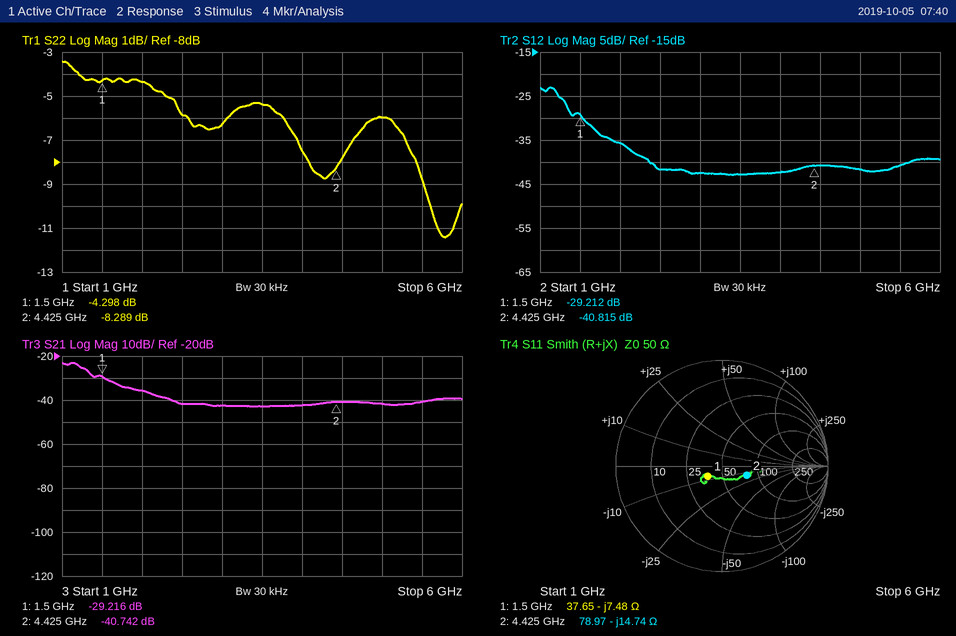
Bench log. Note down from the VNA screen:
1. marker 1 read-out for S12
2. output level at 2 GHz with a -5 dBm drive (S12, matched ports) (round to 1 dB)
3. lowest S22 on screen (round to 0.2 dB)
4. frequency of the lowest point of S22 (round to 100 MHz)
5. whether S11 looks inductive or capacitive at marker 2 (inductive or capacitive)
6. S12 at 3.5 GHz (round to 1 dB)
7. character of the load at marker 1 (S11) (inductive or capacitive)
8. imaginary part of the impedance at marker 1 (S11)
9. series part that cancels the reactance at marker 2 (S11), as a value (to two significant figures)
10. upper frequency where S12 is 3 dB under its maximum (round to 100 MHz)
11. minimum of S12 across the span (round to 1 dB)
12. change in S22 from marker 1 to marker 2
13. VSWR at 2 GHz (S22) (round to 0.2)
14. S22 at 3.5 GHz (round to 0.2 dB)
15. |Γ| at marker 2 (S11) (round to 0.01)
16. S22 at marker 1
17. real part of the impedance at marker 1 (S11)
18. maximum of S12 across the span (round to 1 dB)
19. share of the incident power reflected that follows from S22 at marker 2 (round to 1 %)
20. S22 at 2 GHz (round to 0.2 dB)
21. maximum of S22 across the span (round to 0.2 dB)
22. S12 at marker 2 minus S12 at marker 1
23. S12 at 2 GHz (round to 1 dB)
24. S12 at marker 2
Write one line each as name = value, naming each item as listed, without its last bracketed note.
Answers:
marker 1 read-out for S12 = -29.212 dB
output level at 2 GHz with a -5 dBm drive (S12, matched ports) = -41 dBm
lowest S22 on screen = -11.4 dB
frequency of the lowest point of S22 = 5.8 GHz
whether S11 looks inductive or capacitive at marker 2 = capacitive
S12 at 3.5 GHz = -43 dB
character of the load at marker 1 (S11) = capacitive
imaginary part of the impedance at marker 1 = -7.48 Ω
series part that cancels the reactance at marker 2 (S11), as a value = 530 pH
upper frequency where S12 is 3 dB under its maximum = 1.3 GHz
minimum of S12 across the span = -43 dB
change in S22 from marker 1 to marker 2 = -3.991 dB
VSWR at 2 GHz (S22) = 4.0
S22 at 3.5 GHz = -5.4 dB
|Γ| at marker 2 (S11) = 0.25
S22 at marker 1 = -4.298 dB
real part of the impedance at marker 1 = 37.65 Ω
maximum of S12 across the span = -23 dB
share of the incident power reflected that follows from S22 at marker 2 = 15 %
S22 at 2 GHz = -4.4 dB
maximum of S22 across the span = -3.4 dB
S12 at marker 2 minus S12 at marker 1 = -11.603 dB
S12 at 2 GHz = -36 dB
S12 at marker 2 = -40.815 dB
